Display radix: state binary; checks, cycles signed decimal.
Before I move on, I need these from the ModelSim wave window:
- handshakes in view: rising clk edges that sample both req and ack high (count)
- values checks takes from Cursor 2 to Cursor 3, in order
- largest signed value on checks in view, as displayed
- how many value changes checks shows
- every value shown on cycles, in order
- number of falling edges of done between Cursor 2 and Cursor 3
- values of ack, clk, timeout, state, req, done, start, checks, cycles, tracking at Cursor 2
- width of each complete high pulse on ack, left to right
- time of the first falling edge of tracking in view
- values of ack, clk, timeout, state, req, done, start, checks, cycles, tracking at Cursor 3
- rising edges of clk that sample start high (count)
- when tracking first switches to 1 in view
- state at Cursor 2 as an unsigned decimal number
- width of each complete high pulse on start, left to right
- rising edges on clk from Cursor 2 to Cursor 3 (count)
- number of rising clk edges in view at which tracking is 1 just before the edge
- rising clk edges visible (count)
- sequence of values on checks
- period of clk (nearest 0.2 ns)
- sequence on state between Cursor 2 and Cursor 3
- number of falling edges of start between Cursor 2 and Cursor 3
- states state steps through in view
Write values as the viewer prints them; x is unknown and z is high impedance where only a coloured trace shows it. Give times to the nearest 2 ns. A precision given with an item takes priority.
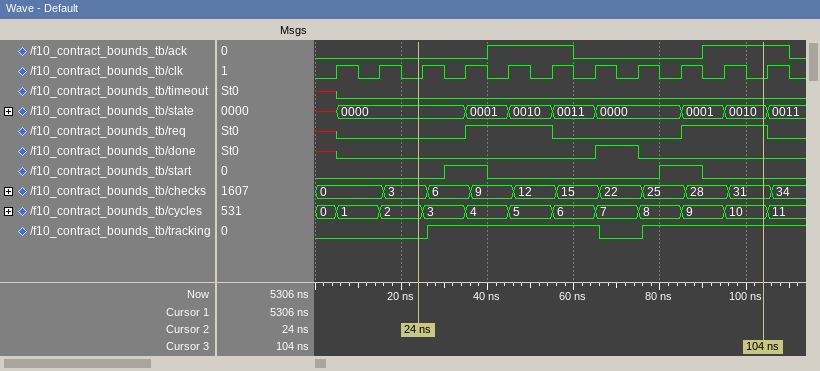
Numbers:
4
3, 6, 9, 12, 15, 22, 25, 28, 31
34
10
0, 1, 2, 3, 4, 5, 6, 7, 8, 9, 10, 11
1
ack=0, clk=0, timeout=0, state=0000, req=0, done=0, start=0, checks=3, cycles=2, tracking=0
20 ns, 20 ns
66 ns
ack=1, clk=0, timeout=0, state=0010, req=1, done=0, start=0, checks=31, cycles=10, tracking=1
2
26 ns
0
10 ns, 10 ns
8
7
11
0, 3, 6, 9, 12, 15, 22, 25, 28, 31, 34
10 ns
0000, 0001, 0010, 0011, 0000, 0001, 0010
2
x, 0000, 0001, 0010, 0011, 0000, 0001, 0010, 0011
